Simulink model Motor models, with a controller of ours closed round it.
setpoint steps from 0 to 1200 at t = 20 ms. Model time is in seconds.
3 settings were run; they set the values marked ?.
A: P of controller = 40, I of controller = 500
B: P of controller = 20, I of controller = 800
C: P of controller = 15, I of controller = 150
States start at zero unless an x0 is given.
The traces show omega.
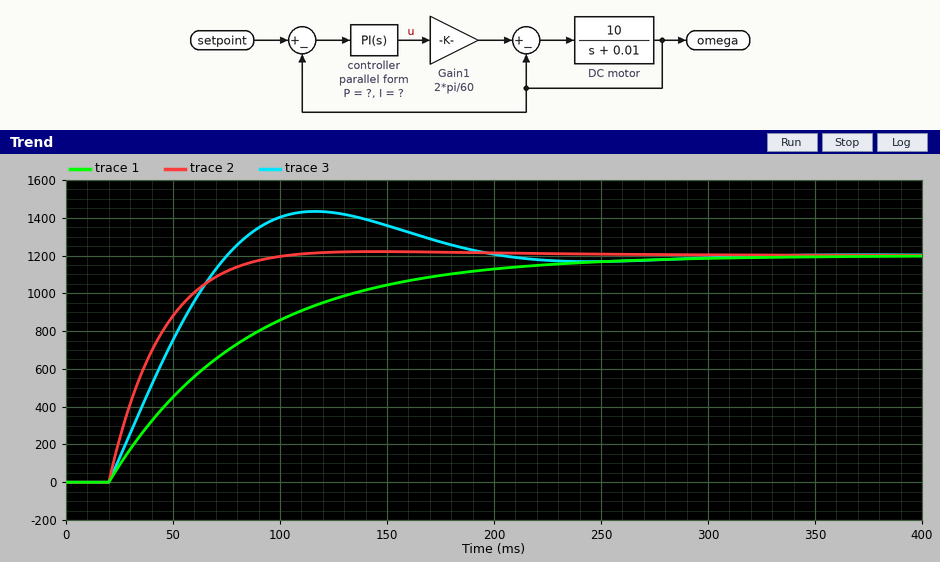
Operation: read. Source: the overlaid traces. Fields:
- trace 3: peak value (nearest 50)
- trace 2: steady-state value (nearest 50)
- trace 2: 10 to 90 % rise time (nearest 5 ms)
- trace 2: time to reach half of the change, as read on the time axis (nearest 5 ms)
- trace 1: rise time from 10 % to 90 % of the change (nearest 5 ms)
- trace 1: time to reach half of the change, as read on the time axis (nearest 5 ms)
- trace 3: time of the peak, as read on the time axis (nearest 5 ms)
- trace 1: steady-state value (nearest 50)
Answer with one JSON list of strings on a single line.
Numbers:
["1450", "1200", "45 ms", "35 ms", "140 ms", "65 ms", "115 ms", "1200"]
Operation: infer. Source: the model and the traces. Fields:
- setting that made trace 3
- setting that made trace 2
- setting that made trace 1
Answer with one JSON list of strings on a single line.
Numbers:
["B", "A", "C"]
